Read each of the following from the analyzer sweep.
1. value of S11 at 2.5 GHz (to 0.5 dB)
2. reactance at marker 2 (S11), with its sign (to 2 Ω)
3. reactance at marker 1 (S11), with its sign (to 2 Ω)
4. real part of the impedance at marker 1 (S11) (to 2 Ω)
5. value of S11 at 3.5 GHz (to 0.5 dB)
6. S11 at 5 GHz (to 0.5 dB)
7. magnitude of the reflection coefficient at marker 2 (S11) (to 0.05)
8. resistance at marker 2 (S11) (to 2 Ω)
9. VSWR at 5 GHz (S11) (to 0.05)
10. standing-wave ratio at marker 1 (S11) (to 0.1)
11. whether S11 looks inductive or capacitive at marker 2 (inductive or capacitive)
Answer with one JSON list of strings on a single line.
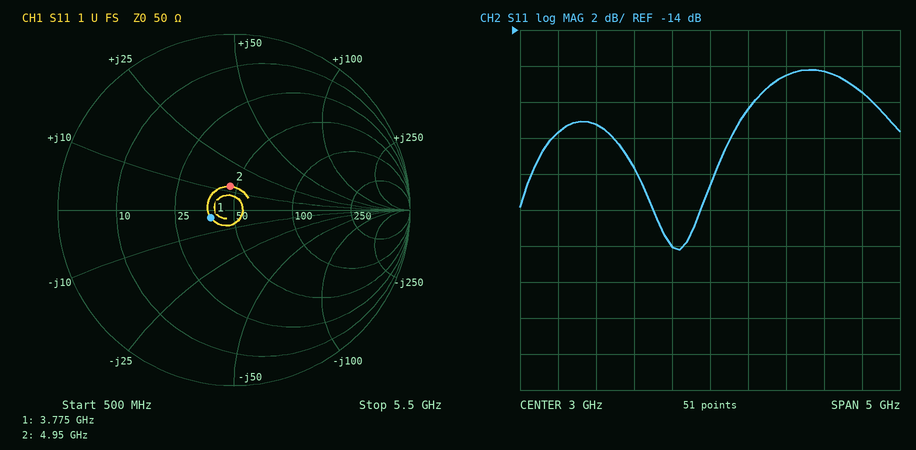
["-26.0 dB", "+12 Ω", "-4 Ω", "38 Ω", "-18.5 dB", "-17.5 dB", "0.15", "46 Ω", "1.30", "1.3", "inductive"]
